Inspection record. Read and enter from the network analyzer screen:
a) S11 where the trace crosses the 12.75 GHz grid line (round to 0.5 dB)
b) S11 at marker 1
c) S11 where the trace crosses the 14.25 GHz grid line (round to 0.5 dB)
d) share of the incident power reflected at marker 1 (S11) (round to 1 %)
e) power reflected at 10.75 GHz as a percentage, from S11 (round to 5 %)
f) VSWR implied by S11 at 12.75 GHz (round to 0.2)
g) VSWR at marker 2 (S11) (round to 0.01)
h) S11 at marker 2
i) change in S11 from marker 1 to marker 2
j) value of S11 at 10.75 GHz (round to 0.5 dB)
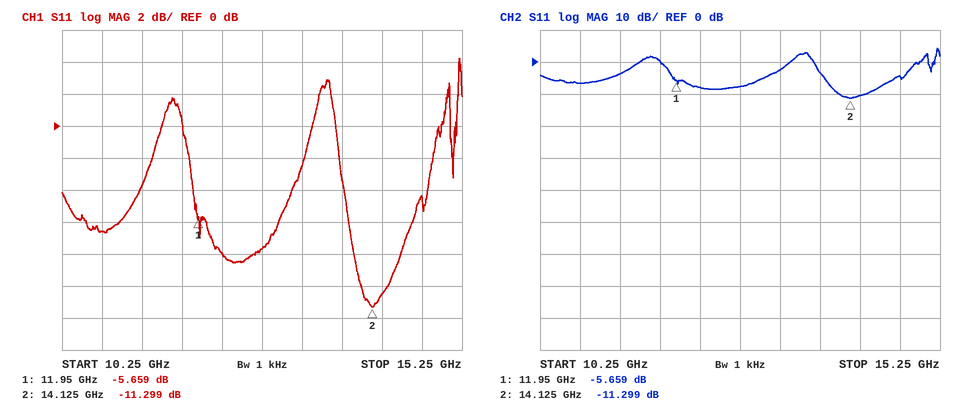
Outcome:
-7.5 dB
-5.659 dB
-10.5 dB
27 %
20 %
2.4
1.75
-11.299 dB
-5.640 dB
-6.5 dB
